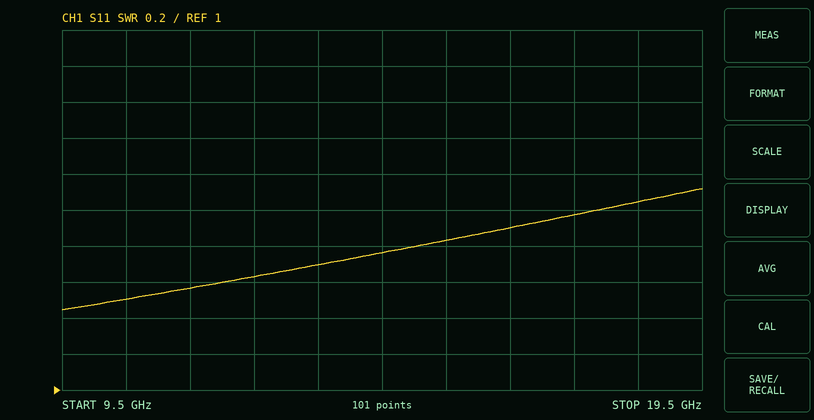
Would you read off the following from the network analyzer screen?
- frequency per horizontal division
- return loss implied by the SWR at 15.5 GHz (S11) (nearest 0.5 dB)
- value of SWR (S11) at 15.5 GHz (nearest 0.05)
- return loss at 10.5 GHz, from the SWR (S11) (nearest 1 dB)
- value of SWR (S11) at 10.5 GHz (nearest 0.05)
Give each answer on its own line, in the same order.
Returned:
1 GHz
10.5 dB
1.85
14 dB
1.50
